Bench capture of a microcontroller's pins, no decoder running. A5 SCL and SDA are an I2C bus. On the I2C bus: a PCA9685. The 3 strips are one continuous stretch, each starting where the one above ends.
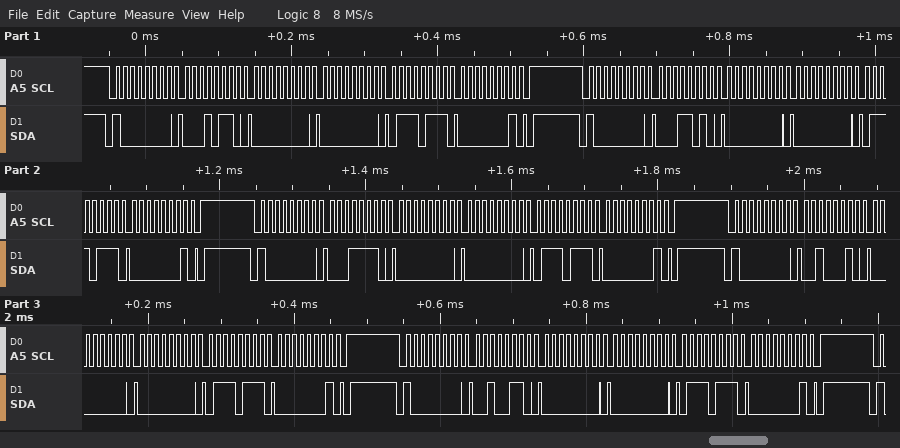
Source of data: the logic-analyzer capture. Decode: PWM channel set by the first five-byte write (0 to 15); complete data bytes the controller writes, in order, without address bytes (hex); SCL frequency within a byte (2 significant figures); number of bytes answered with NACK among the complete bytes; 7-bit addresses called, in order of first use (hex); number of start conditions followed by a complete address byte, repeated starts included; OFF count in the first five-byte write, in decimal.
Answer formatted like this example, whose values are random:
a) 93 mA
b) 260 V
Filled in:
a) 4
b) 16 00 00 77 01 1A 00 00 77 01 1E 00 00 77 01 22 00 00 77 01 26 00 00 77 01
c) 100 kHz
d) 0
e) 0x40
f) 5
g) 375
